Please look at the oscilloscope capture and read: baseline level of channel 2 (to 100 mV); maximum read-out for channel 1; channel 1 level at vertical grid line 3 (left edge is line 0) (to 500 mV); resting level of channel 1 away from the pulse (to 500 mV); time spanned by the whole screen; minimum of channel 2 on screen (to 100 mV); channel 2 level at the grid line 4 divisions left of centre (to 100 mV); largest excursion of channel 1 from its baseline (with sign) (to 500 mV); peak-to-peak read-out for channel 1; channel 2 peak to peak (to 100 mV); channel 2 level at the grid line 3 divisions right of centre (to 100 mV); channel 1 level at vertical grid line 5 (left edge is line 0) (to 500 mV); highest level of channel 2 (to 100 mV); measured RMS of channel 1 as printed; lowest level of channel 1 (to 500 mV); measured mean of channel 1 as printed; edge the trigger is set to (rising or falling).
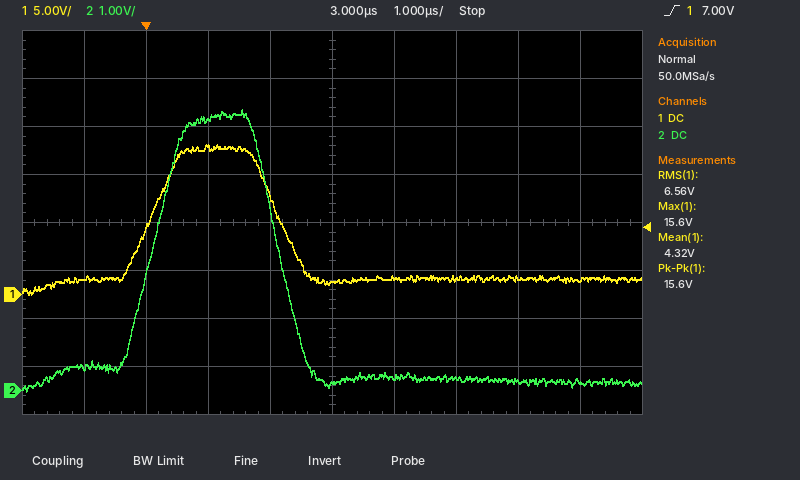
200 mV
15.6 V
15.5 V
1.5 V
10 µs
0.0 V
500 mV
+14.0 V
15.6 V
5.9 V
200 mV
1.0 V
5.9 V
6.56 V
0.0 V
4.32 V
rising
